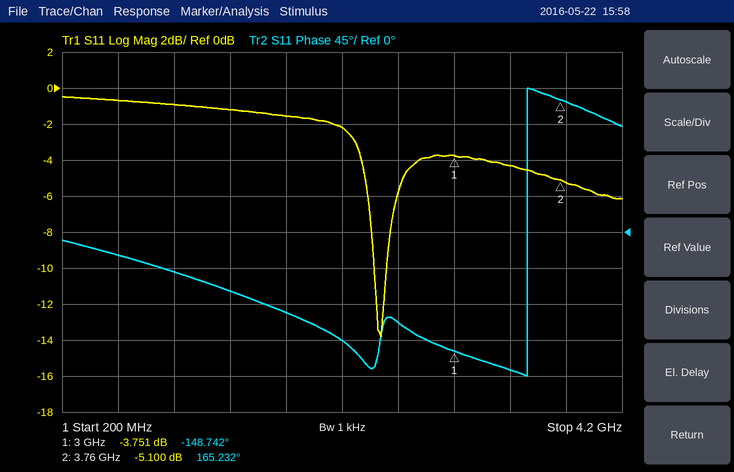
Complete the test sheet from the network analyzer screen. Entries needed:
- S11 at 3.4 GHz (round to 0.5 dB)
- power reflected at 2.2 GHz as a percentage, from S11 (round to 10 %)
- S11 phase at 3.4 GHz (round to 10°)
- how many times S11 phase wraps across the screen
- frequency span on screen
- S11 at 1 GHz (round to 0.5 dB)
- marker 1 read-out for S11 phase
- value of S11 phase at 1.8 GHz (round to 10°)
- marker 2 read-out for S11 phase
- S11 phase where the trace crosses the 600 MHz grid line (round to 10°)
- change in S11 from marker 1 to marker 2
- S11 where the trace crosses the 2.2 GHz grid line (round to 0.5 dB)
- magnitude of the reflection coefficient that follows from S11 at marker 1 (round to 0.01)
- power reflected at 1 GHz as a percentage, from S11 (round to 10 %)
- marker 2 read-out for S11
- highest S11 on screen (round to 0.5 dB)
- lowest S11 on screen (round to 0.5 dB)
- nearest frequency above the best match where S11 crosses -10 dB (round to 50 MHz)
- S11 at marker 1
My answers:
-4.5 dB
60 %
-170°
1
4 GHz
-1.0 dB
-148.742°
-100°
165.232°
-30°
-1.349 dB
-2.0 dB
0.65
80 %
-5.100 dB
-0.5 dB
-14.0 dB
2.50 GHz
-3.751 dB
